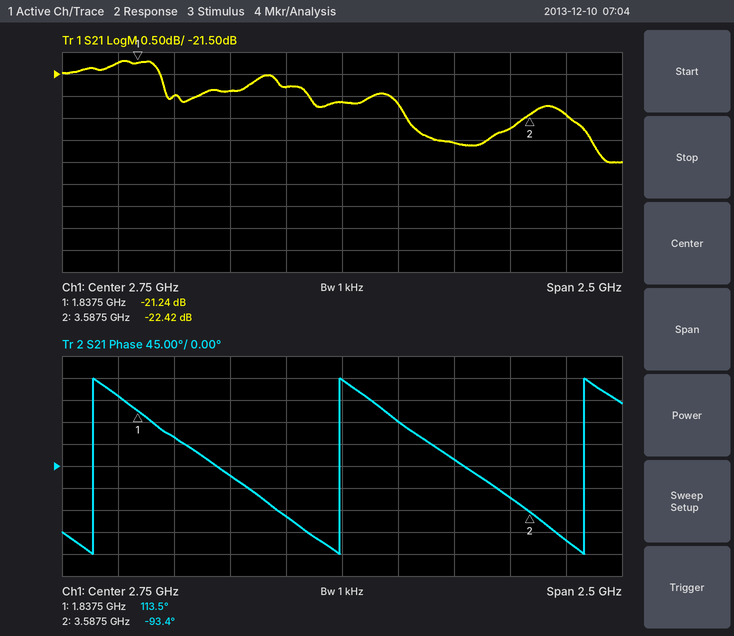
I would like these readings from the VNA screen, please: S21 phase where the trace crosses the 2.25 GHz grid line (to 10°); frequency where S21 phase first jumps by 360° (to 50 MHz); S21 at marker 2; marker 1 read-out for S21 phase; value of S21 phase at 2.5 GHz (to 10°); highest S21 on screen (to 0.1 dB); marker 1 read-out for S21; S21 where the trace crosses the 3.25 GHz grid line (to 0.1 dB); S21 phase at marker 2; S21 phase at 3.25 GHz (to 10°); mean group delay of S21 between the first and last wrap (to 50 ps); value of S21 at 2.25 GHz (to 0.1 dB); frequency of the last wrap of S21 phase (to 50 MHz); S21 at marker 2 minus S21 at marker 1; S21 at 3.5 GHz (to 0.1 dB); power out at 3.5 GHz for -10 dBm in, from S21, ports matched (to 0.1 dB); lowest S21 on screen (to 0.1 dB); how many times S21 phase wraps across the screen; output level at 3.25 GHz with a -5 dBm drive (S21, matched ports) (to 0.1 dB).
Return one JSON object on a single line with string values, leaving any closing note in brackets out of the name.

{"S21 phase where the trace crosses the 2.25 GHz grid line": "-20°", "frequency where S21 phase first jumps by 360°": "1.65 GHz", "S21 at marker 2": "-22.42 dB", "marker 1 read-out for S21 phase": "113.5°", "value of S21 phase at 2.5 GHz": "-100°", "highest S21 on screen": "-21.2 dB", "marker 1 read-out for S21": "-21.24 dB", "S21 where the trace crosses the 3.25 GHz grid line": "-23.1 dB", "S21 phase at marker 2": "-93.4°", "S21 phase at 3.25 GHz": "10°", "mean group delay of S21 between the first and last wrap": "900 ps", "value of S21 at 2.25 GHz": "-21.9 dB", "frequency of the last wrap of S21 phase": "3.85 GHz", "S21 at marker 2 minus S21 at marker 1": "-1.18 dB", "S21 at 3.5 GHz": "-22.7 dB", "power out at 3.5 GHz for -10 dBm in, from S21, ports matched": "-32.7 dBm", "lowest S21 on screen": "-23.5 dB", "how many times S21 phase wraps across the screen": "3", "output level at 3.25 GHz with a -5 dBm drive (S21, matched ports)": "-28.1 dBm"}
